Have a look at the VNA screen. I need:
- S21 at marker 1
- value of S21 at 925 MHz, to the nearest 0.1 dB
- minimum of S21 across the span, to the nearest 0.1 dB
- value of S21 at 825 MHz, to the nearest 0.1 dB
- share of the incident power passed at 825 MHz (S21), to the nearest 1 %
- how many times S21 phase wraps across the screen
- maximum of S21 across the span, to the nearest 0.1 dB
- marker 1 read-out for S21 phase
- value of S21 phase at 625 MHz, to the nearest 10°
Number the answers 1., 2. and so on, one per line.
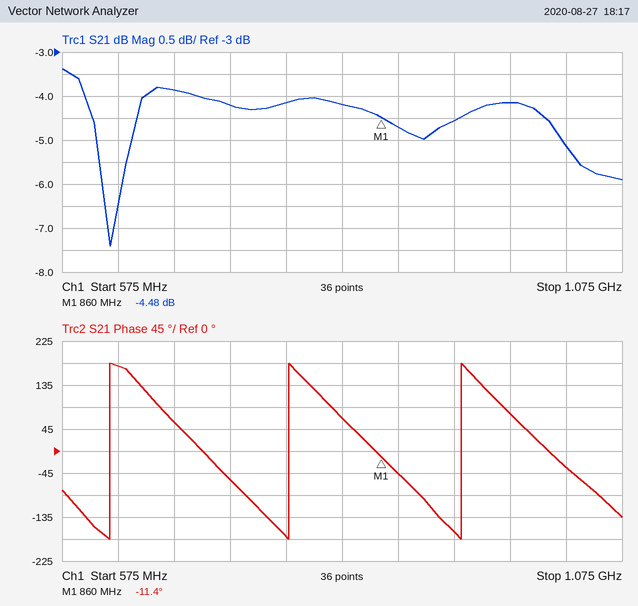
1. -4.48 dB
2. -4.6 dB
3. -7.4 dB
4. -4.2 dB
5. 38 %
6. 3
7. -3.4 dB
8. -11.4°
9. 170°
